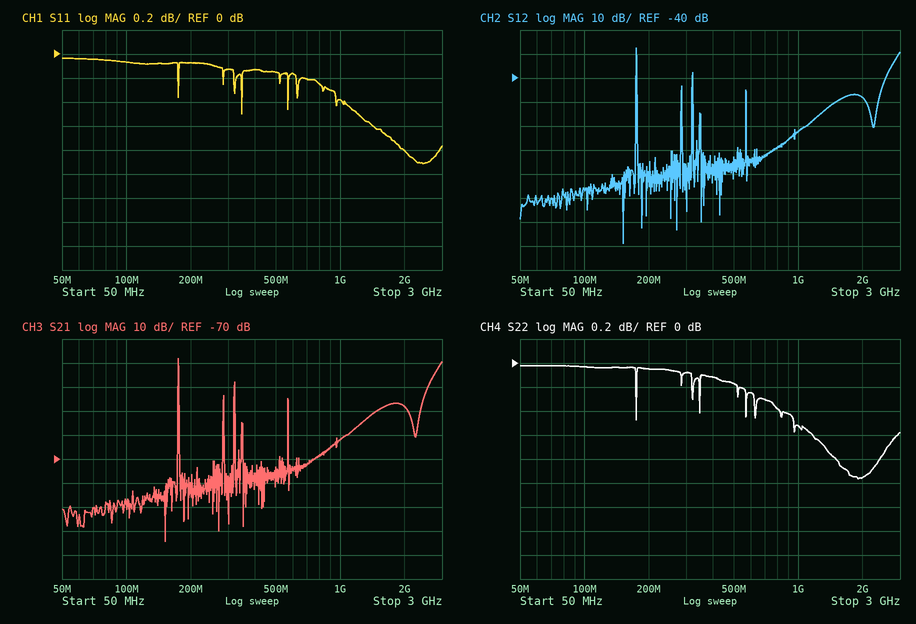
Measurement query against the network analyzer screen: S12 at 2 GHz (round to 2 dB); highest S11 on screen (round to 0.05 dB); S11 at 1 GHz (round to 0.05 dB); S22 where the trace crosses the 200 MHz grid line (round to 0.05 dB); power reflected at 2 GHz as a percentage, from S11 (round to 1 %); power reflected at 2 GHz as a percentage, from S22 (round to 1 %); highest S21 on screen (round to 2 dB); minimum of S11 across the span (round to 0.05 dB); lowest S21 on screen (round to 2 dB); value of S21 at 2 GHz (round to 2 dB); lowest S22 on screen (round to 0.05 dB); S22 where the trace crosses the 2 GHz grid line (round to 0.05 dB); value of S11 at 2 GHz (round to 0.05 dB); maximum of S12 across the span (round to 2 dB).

-48 dB
-0.05 dB
-0.40 dB
-0.05 dB
83 %
80 %
-28 dB
-0.90 dB
-104 dB
-48 dB
-0.95 dB
-0.95 dB
-0.80 dB
-28 dB
